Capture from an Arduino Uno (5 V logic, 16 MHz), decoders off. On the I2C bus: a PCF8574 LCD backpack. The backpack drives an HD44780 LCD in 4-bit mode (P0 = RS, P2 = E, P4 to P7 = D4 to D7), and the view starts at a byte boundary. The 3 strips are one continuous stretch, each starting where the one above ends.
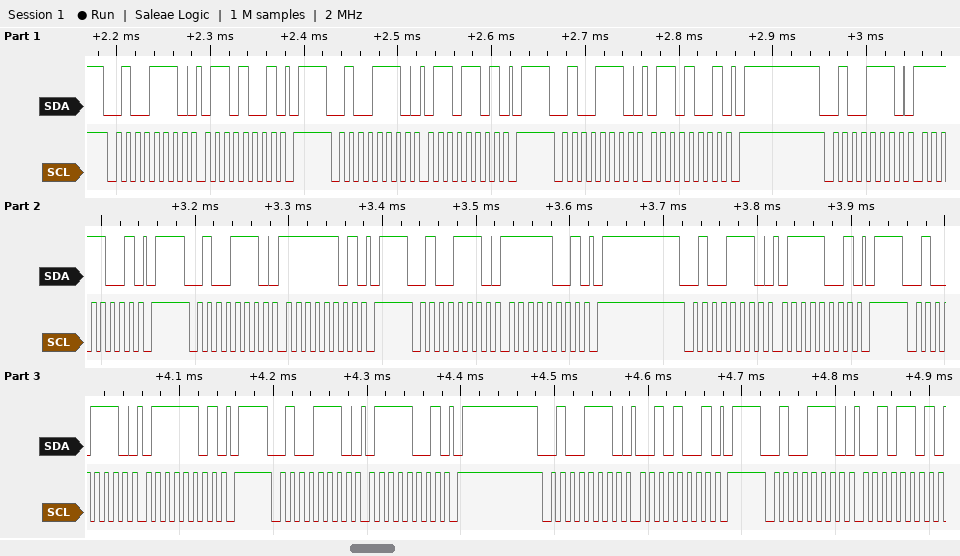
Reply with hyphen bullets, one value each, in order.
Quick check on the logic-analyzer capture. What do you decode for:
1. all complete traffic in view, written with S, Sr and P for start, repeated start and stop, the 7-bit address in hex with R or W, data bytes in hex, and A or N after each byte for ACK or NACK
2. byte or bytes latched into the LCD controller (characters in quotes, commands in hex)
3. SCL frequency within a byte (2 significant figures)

- S 27W A 69 A P S 27W A 6D A P S 27W A 69 A P S 27W A F9 A P S 27W A FD A P S 27W A F9 A P S 27W A 79 A P S 27W A 7D A P S 27W A 79 A P S 27W A 29 A P S 27W A 2D A
- 'o'
- 100 kHz
